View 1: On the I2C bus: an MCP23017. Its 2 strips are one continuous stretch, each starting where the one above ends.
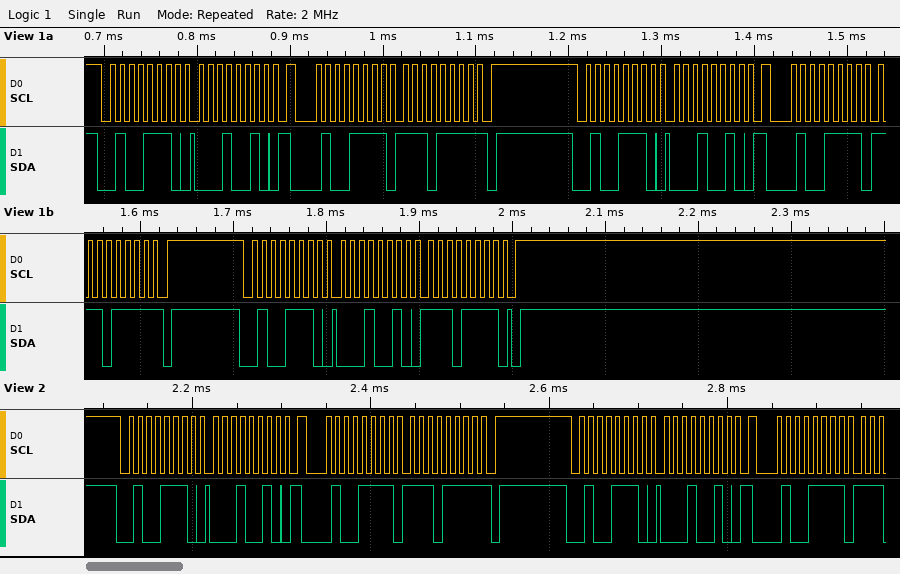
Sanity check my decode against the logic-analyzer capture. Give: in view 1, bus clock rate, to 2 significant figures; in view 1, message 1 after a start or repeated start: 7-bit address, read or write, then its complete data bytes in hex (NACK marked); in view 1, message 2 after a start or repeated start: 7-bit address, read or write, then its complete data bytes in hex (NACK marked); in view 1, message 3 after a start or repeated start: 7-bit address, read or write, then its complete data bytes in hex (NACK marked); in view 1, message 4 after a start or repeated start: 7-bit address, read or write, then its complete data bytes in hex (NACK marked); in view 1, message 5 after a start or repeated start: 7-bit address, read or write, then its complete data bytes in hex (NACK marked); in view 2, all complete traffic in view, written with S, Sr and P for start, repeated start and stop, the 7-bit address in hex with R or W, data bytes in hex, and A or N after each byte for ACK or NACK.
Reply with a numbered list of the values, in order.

1. 100 kHz
2. 0x27 write: 12
3. 0x27 read: EF NACK
4. 0x27 write: 12
5. 0x27 read: EF NACK
6. 0x27 write: 12 EF
7. S 27W A 12 A Sr 27R A EF N P S 27W A 12 A Sr 27R A
